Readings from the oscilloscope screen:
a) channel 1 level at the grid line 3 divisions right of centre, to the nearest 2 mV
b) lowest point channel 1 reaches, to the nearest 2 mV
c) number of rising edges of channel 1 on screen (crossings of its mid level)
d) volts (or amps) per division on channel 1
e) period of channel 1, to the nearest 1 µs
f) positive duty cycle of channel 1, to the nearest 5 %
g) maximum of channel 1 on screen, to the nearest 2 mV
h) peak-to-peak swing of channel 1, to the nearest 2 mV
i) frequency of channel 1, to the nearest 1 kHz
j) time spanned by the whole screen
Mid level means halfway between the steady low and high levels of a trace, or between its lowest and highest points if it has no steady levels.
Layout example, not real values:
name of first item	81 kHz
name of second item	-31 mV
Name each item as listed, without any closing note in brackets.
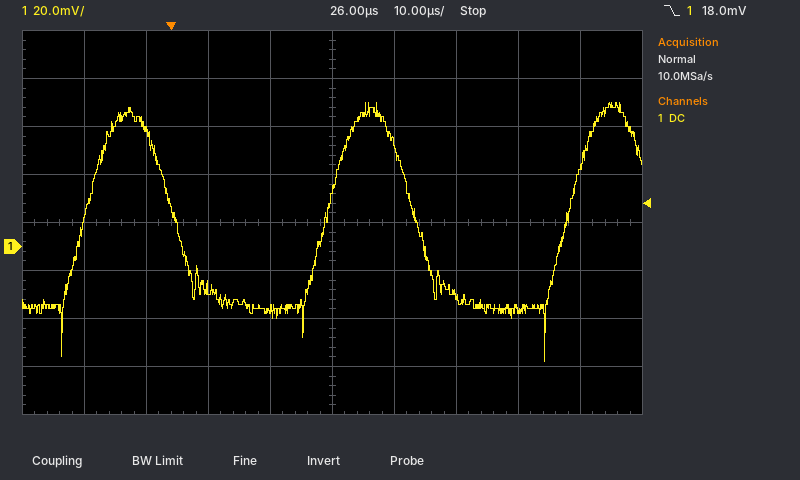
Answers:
channel 1 level at the grid line 3 divisions right of centre, to the nearest 2 mV	-26 mV
lowest point channel 1 reaches, to the nearest 2 mV	-48 mV
number of rising edges of channel 1 on screen	3
volts (or amps) per division on channel 1	20 mV
period of channel 1, to the nearest 1 µs	39 µs
positive duty cycle of channel 1, to the nearest 5 %	40 %
maximum of channel 1 on screen, to the nearest 2 mV	60 mV
peak-to-peak swing of channel 1, to the nearest 2 mV	108 mV
frequency of channel 1, to the nearest 1 kHz	26 kHz
time spanned by the whole screen	100 µs
